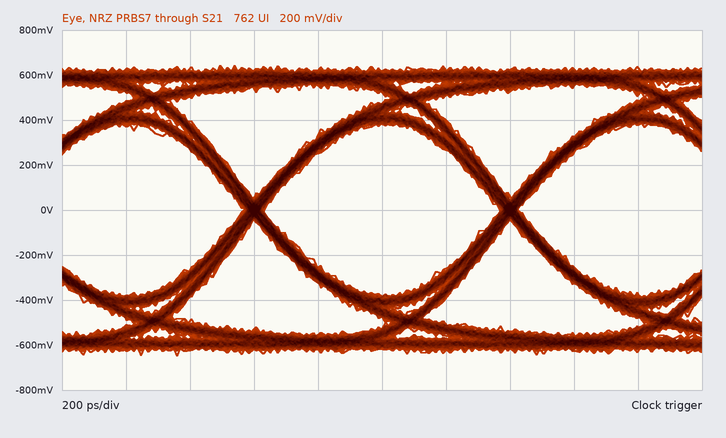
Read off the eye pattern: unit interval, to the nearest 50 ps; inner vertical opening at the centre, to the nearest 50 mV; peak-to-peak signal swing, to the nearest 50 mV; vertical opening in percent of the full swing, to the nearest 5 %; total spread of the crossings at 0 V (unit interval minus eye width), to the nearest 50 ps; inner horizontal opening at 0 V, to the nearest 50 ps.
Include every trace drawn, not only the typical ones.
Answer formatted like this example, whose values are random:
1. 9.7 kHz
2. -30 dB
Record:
1. 800 ps
2. 750 mV
3. 1.30 V
4. 60 %
5. 50 ps
6. 750 ps
